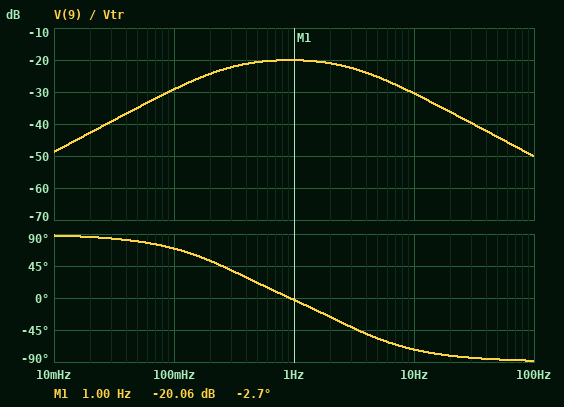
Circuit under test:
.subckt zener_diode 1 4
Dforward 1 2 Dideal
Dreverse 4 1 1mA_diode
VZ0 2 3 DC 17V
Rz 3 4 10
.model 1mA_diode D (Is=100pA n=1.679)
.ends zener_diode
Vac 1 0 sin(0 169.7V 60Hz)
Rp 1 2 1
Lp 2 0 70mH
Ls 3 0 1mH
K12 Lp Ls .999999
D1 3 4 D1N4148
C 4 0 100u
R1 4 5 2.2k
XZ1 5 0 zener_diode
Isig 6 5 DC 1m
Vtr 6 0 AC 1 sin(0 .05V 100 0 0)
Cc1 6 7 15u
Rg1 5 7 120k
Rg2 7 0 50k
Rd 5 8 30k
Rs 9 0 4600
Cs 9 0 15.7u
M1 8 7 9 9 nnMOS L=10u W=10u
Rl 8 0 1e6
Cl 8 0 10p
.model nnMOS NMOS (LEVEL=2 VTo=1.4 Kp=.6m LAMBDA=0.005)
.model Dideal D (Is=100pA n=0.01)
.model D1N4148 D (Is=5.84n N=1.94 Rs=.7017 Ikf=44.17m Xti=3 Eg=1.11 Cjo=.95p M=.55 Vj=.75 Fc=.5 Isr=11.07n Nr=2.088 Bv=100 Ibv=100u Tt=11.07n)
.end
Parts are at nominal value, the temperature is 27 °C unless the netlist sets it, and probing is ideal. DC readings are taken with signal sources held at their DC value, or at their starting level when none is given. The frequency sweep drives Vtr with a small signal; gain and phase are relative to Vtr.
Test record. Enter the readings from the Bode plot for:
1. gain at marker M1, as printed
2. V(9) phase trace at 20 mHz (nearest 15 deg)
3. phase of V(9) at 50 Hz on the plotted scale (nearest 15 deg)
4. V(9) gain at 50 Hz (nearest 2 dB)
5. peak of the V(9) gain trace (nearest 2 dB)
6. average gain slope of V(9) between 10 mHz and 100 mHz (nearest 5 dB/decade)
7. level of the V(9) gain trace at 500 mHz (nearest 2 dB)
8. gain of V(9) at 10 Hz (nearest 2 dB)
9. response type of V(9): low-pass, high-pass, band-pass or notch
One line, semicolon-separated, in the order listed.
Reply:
-20.06 dB; 90 deg; -90 deg; -44 dB; -20 dB; 20 dB/decade; -20 dB; -30 dB; band-pass
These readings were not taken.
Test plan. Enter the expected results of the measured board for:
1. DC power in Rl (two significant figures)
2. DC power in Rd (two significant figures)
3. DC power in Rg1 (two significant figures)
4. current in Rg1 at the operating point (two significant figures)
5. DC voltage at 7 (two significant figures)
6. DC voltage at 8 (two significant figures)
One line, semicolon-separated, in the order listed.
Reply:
8.2 µW; 6.7 mW; 1.2 mW; 100 µA; 5.0 V; 2.9 V
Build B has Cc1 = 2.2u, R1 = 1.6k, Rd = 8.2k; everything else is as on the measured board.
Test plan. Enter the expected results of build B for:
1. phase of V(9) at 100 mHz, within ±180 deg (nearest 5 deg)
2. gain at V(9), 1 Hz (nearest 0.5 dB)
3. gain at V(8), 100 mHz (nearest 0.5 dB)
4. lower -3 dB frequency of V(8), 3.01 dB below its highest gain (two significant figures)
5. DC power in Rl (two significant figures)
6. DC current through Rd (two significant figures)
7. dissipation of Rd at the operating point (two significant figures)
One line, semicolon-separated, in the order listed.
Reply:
85 deg; -9.5 dB; -23.5 dB; 10 Hz; 160 µW; 520 µA; 2.2 mW
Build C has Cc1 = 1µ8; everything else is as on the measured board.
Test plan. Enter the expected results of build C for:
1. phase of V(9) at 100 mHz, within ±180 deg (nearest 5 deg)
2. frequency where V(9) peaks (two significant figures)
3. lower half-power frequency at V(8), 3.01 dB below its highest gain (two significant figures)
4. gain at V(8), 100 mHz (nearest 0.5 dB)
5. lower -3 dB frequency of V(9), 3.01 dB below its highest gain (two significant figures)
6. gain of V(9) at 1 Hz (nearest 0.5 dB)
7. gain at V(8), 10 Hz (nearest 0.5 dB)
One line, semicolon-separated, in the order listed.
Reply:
85 deg; 2.7 Hz; 3.1 Hz; -31.0 dB; 1.1 Hz; -28.5 dB; -1.5 dB
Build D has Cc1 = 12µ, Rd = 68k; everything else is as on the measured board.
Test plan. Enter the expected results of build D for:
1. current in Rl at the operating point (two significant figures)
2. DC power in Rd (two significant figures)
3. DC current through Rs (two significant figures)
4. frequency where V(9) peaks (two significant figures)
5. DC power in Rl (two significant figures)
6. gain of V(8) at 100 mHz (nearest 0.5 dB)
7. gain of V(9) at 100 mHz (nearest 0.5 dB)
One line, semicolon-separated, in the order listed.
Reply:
1.2 µA; 3.7 mW; 230 µA; 940 mHz; 1.5 µW; -36.0 dB; -59.0 dB
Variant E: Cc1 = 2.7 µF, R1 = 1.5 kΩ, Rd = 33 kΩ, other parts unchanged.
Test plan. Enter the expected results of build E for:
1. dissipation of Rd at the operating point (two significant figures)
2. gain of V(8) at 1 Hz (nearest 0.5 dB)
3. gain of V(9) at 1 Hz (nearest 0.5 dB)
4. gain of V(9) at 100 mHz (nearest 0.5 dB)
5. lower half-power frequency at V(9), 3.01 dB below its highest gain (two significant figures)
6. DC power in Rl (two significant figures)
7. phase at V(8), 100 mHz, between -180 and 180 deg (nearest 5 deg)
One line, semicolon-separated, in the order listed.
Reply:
6.3 mW; -13.5 dB; -31.0 dB; -49.0 dB; 860 mHz; 6.5 µW; -95 deg
